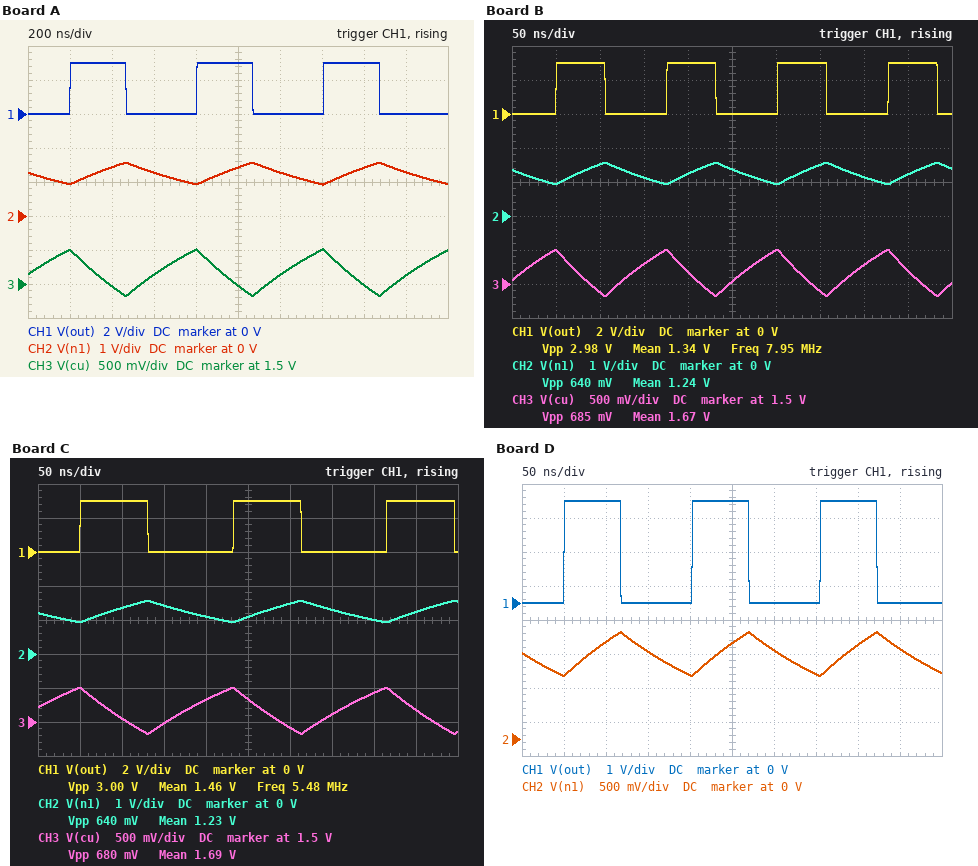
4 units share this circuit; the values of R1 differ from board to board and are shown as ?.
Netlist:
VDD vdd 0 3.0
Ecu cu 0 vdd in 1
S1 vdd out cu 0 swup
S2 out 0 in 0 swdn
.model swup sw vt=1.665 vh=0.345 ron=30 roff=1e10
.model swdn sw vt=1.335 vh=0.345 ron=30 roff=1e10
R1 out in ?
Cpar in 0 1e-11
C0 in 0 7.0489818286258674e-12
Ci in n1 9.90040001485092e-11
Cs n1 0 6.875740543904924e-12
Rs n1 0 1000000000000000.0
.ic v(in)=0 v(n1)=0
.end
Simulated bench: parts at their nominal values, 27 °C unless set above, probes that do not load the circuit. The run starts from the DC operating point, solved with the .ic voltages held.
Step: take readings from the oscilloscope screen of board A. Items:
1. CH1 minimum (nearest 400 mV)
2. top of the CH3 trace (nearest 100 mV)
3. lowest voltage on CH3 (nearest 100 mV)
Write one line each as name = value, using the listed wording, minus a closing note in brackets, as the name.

CH1 minimum = 0 V
top of the CH3 trace = 2.0 V
lowest voltage on CH3 = 1.3 V
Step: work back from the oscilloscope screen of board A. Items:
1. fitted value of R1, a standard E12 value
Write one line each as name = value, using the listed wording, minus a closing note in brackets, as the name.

fitted value of R1, a standard E12 value = 27 kΩ
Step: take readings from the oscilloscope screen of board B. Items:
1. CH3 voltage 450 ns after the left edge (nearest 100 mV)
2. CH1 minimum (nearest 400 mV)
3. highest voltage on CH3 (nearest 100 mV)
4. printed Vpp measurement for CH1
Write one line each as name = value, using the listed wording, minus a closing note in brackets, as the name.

CH3 voltage 450 ns after the left edge = 1.7 V
CH1 minimum = 0 V
highest voltage on CH3 = 2.0 V
printed Vpp measurement for CH1 = 2.98 V
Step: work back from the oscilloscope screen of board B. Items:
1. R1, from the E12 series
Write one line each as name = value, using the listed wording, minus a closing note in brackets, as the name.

R1, from the E12 series = 5.6 kΩ
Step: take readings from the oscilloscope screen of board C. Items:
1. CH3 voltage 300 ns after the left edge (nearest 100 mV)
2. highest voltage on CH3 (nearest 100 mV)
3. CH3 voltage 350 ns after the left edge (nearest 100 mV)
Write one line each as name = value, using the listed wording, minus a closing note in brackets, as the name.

CH3 voltage 300 ns after the left edge = 1.4 V
highest voltage on CH3 = 2.0 V
CH3 voltage 350 ns after the left edge = 1.6 V
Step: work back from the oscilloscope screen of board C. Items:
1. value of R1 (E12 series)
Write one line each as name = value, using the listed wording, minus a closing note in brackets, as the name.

value of R1 = 8.2 kΩ
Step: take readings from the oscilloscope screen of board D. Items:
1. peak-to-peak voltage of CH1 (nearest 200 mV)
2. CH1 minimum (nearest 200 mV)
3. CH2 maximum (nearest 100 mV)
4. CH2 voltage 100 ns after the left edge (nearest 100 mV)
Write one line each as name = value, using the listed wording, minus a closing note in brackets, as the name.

peak-to-peak voltage of CH1 = 3.0 V
CH1 minimum = 0 V
CH2 maximum = 1.6 V
CH2 voltage 100 ns after the left edge = 1.4 V
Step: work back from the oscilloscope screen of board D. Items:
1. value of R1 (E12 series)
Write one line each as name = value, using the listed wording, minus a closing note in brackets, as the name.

value of R1 = 6.8 kΩ
